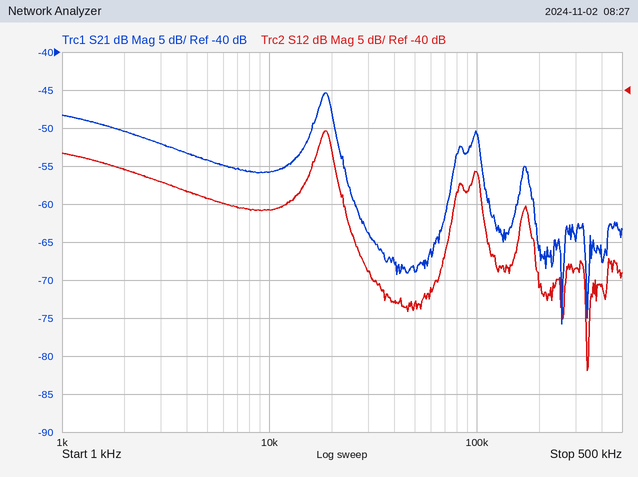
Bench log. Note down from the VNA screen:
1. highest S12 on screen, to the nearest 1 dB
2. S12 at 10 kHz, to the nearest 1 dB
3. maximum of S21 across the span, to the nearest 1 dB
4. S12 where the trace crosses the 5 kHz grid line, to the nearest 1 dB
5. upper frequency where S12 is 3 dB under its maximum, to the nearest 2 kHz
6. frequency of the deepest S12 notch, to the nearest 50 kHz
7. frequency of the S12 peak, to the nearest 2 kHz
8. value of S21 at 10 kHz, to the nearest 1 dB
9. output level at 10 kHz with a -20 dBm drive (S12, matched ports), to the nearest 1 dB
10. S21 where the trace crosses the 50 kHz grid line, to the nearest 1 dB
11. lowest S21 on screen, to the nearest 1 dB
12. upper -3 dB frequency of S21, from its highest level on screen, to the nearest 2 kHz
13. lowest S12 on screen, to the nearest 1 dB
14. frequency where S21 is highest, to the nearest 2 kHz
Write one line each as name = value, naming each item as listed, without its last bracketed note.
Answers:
highest S12 on screen, to the nearest 1 dB = -45 dB
S12 at 10 kHz, to the nearest 1 dB = -56 dB
maximum of S21 across the span, to the nearest 1 dB = -45 dB
S12 where the trace crosses the 5 kHz grid line, to the nearest 1 dB = -54 dB
upper frequency where S12 is 3 dB under its maximum, to the nearest 2 kHz = 20 kHz
frequency of the deepest S12 notch, to the nearest 50 kHz = 350 kHz
frequency of the S12 peak, to the nearest 2 kHz = 18 kHz
value of S21 at 10 kHz, to the nearest 1 dB = -56 dB
output level at 10 kHz with a -20 dBm drive (S12, matched ports), to the nearest 1 dB = -76 dBm
S21 where the trace crosses the 50 kHz grid line, to the nearest 1 dB = -69 dB
lowest S21 on screen, to the nearest 1 dB = -76 dB
upper -3 dB frequency of S21, from its highest level on screen, to the nearest 2 kHz = 20 kHz
lowest S12 on screen, to the nearest 1 dB = -77 dB
frequency where S21 is highest, to the nearest 2 kHz = 18 kHz
